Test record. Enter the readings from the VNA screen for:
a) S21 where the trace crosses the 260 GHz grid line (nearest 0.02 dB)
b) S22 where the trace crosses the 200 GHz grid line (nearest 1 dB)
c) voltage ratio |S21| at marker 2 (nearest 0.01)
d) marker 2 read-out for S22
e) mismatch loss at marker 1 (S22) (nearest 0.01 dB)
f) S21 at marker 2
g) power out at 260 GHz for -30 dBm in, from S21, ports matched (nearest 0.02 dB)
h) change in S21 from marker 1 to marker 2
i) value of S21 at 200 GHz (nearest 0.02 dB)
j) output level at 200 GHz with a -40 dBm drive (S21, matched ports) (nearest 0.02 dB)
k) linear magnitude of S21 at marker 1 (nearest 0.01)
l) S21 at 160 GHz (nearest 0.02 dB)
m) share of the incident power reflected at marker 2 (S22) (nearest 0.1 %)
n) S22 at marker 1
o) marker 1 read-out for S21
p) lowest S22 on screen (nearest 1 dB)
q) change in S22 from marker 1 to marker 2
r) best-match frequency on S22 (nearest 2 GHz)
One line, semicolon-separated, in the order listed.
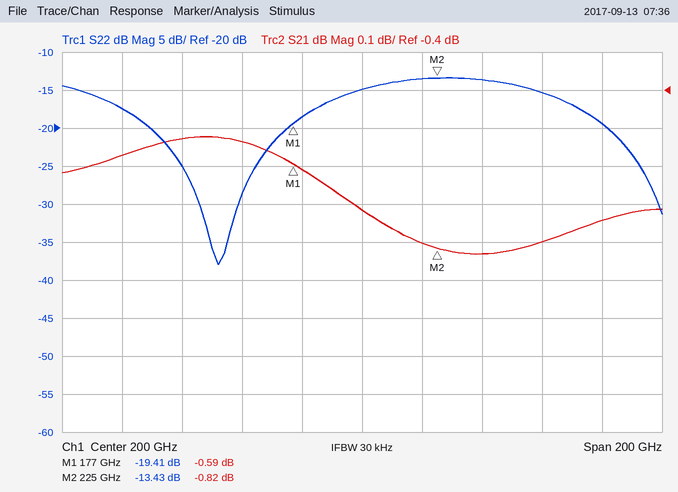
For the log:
-0.80 dB; -15 dB; 0.91; -13.43 dB; 0.05 dB; -0.82 dB; -30.80 dBm; -0.23 dB; -0.72 dB; -40.72 dBm; 0.93; -0.54 dB; 4.5 %; -19.41 dB; -0.59 dB; -38 dB; 5.98 dB; 152 GHz
